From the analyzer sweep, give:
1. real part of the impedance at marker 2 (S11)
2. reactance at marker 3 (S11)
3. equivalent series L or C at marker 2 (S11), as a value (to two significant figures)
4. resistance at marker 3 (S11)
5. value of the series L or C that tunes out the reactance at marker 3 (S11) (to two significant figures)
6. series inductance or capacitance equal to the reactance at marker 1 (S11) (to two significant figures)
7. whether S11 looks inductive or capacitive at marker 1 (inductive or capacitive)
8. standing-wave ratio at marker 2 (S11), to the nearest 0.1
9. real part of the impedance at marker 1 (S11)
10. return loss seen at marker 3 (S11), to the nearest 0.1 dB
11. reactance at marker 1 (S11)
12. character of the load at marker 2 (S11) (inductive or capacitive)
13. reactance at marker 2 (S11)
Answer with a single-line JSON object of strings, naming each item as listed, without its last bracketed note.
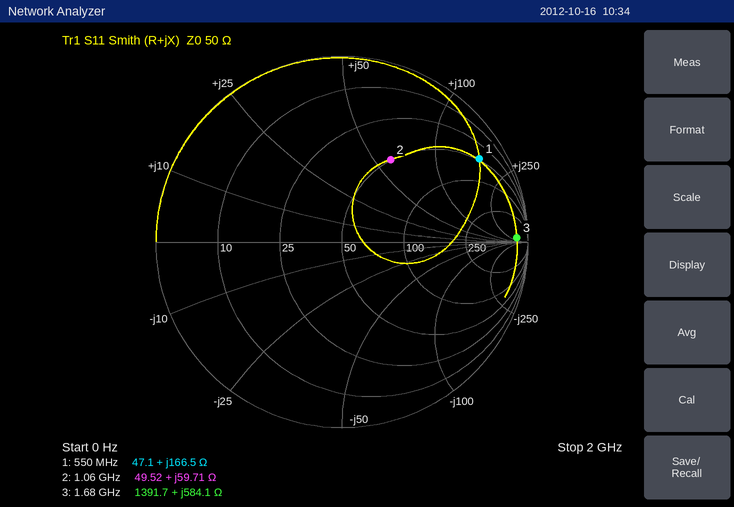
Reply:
{"real part of the impedance at marker 2": "49.52 Ω", "reactance at marker 3": "+584.1 Ω", "equivalent series L or C at marker 2 (S11), as a value": "9.0 nH", "resistance at marker 3": "1391.7 Ω", "value of the series L or C that tunes out the reactance at marker 3 (S11)": "160 fF", "series inductance or capacitance equal to the reactance at marker 1 (S11)": "48 nH", "whether S11 looks inductive or capacitive at marker 1": "inductive", "standing-wave ratio at marker 2 (S11), to the nearest 0.1": "3.1", "real part of the impedance at marker 1": "47.1 Ω", "return loss seen at marker 3 (S11), to the nearest 0.1 dB": "0.5 dB", "reactance at marker 1": "+166.5 Ω", "character of the load at marker 2 (S11)": "inductive", "reactance at marker 2": "+59.71 Ω"}
